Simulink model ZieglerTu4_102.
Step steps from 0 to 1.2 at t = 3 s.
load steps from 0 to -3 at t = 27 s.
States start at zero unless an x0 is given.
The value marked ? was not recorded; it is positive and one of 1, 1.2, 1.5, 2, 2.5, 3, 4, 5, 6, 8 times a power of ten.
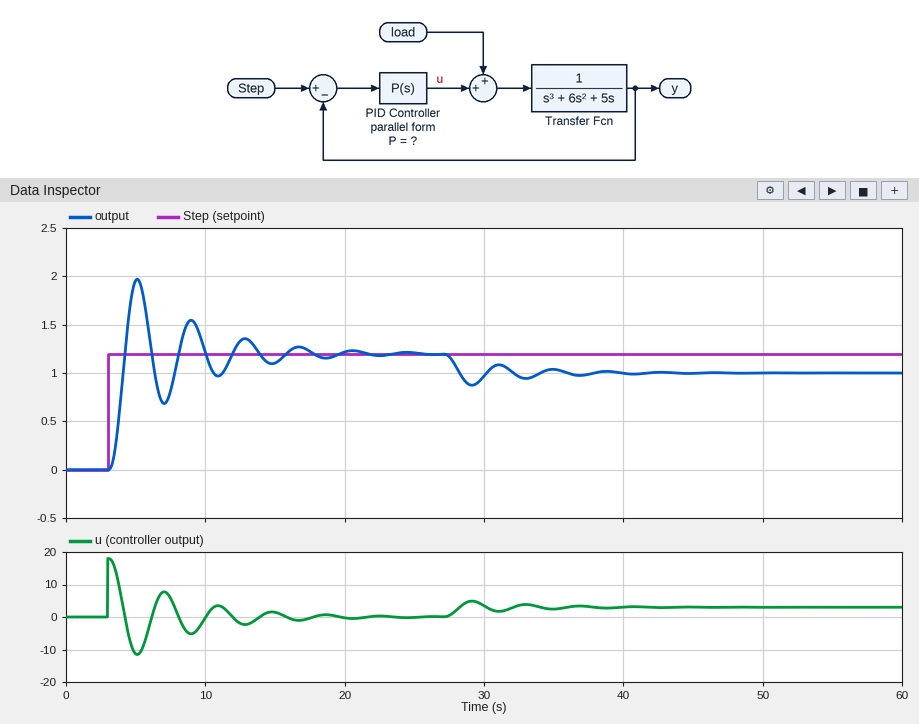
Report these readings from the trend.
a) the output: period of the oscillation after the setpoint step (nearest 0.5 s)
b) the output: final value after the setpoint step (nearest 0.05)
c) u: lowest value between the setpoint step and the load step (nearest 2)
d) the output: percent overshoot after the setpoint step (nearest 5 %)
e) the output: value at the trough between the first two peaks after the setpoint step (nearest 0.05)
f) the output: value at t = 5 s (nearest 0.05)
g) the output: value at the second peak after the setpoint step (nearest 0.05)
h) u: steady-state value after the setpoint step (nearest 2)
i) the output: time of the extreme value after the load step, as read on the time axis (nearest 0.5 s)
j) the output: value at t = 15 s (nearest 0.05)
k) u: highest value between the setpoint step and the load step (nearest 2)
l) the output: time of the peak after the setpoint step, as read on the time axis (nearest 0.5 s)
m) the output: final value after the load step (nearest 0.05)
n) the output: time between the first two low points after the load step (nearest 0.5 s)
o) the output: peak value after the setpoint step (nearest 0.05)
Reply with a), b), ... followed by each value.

a) 4.0 s
b) 1.20
c) -12
d) 65 %
e) 0.70
f) 1.95
g) 1.55
h) 0
i) 29.0 s
j) 1.10
k) 18
l) 5.0 s
m) 1.00
n) 4.0 s
o) 1.95
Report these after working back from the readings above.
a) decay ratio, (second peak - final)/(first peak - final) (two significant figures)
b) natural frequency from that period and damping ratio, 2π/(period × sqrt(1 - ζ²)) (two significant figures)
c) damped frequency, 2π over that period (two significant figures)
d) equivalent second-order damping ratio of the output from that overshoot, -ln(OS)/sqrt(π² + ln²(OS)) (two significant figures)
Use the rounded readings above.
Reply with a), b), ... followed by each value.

a) 0.47
b) 1.6 rad/s
c) 1.6 rad/s
d) 0.14
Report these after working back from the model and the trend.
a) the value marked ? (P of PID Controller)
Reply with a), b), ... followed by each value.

a) 15
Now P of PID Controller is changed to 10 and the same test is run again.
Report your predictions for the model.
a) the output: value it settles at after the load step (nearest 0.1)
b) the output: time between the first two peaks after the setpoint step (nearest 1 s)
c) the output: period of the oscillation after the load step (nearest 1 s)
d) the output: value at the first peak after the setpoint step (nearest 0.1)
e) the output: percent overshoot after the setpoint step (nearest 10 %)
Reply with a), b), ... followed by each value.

a) 0.9
b) 5 s
c) 5 s
d) 1.8
e) 50 %
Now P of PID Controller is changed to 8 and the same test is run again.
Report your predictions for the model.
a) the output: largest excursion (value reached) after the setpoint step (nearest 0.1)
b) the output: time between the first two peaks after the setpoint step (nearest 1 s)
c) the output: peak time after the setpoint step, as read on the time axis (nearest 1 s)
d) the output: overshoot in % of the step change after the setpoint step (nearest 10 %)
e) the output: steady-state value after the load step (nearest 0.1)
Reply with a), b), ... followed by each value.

a) 1.7
b) 5 s
c) 6 s
d) 40 %
e) 0.8
